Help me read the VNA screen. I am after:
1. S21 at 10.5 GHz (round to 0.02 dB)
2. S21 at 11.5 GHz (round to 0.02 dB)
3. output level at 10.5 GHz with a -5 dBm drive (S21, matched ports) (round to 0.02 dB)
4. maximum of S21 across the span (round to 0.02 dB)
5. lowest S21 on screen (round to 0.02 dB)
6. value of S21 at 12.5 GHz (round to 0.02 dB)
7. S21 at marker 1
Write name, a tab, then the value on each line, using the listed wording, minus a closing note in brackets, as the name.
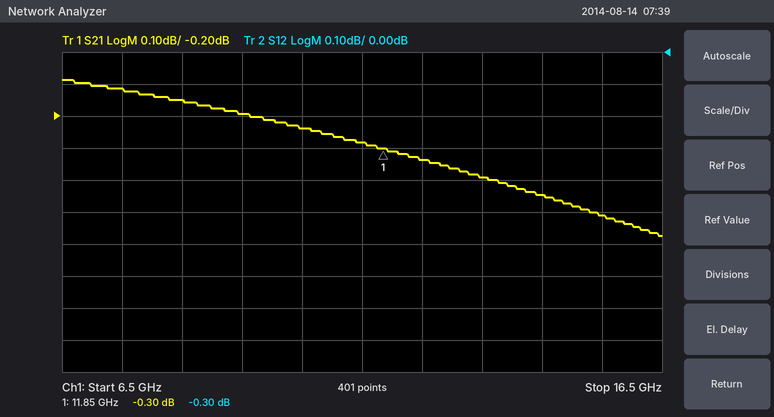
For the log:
S21 at 10.5 GHz	-0.24 dB
S21 at 11.5 GHz	-0.28 dB
output level at 10.5 GHz with a -5 dBm drive (S21, matched ports)	-5.24 dBm
maximum of S21 across the span	-0.08 dB
lowest S21 on screen	-0.58 dB
value of S21 at 12.5 GHz	-0.34 dB
S21 at marker 1	-0.30 dB
